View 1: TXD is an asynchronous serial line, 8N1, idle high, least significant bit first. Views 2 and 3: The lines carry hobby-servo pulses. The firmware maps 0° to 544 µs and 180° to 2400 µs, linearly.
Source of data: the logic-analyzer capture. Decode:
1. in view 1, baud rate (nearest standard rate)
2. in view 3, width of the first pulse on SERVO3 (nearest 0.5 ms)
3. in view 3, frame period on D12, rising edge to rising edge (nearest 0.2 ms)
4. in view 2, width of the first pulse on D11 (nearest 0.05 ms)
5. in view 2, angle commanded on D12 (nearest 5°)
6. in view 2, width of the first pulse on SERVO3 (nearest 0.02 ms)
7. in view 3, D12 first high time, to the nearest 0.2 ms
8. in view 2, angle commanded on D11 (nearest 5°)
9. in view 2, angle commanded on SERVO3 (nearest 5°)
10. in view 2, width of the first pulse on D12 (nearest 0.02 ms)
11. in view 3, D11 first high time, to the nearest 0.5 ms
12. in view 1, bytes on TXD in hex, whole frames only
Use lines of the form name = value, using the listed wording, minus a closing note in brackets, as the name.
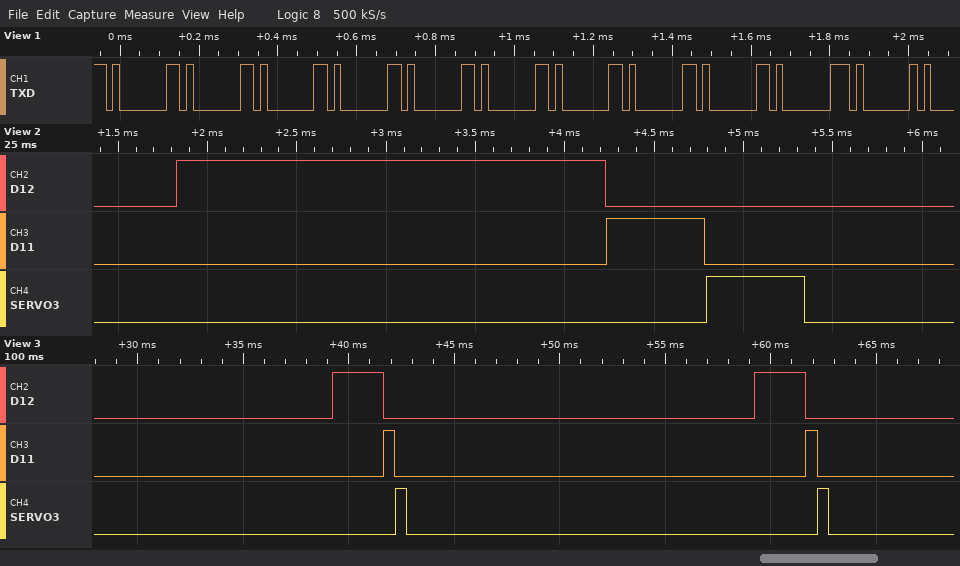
in view 1, baud rate = 57600 baud
in view 3, width of the first pulse on SERVO3 = 0.5 ms
in view 3, frame period on D12, rising edge to rising edge = 20.0 ms
in view 2, width of the first pulse on D11 = 0.55 ms
in view 2, angle commanded on D12 = 180°
in view 2, width of the first pulse on SERVO3 = 0.54 ms
in view 3, D12 first high time, to the nearest 0.2 ms = 2.4 ms
in view 2, angle commanded on D11 = 0°
in view 2, angle commanded on SERVO3 = 0°
in view 2, width of the first pulse on D12 = 2.40 ms
in view 3, D11 first high time, to the nearest 0.5 ms = 0.5 ms
in view 1, bytes on TXD in hex, whole frames only = 01 01 01 01 01 01 01 01 01 01 01
